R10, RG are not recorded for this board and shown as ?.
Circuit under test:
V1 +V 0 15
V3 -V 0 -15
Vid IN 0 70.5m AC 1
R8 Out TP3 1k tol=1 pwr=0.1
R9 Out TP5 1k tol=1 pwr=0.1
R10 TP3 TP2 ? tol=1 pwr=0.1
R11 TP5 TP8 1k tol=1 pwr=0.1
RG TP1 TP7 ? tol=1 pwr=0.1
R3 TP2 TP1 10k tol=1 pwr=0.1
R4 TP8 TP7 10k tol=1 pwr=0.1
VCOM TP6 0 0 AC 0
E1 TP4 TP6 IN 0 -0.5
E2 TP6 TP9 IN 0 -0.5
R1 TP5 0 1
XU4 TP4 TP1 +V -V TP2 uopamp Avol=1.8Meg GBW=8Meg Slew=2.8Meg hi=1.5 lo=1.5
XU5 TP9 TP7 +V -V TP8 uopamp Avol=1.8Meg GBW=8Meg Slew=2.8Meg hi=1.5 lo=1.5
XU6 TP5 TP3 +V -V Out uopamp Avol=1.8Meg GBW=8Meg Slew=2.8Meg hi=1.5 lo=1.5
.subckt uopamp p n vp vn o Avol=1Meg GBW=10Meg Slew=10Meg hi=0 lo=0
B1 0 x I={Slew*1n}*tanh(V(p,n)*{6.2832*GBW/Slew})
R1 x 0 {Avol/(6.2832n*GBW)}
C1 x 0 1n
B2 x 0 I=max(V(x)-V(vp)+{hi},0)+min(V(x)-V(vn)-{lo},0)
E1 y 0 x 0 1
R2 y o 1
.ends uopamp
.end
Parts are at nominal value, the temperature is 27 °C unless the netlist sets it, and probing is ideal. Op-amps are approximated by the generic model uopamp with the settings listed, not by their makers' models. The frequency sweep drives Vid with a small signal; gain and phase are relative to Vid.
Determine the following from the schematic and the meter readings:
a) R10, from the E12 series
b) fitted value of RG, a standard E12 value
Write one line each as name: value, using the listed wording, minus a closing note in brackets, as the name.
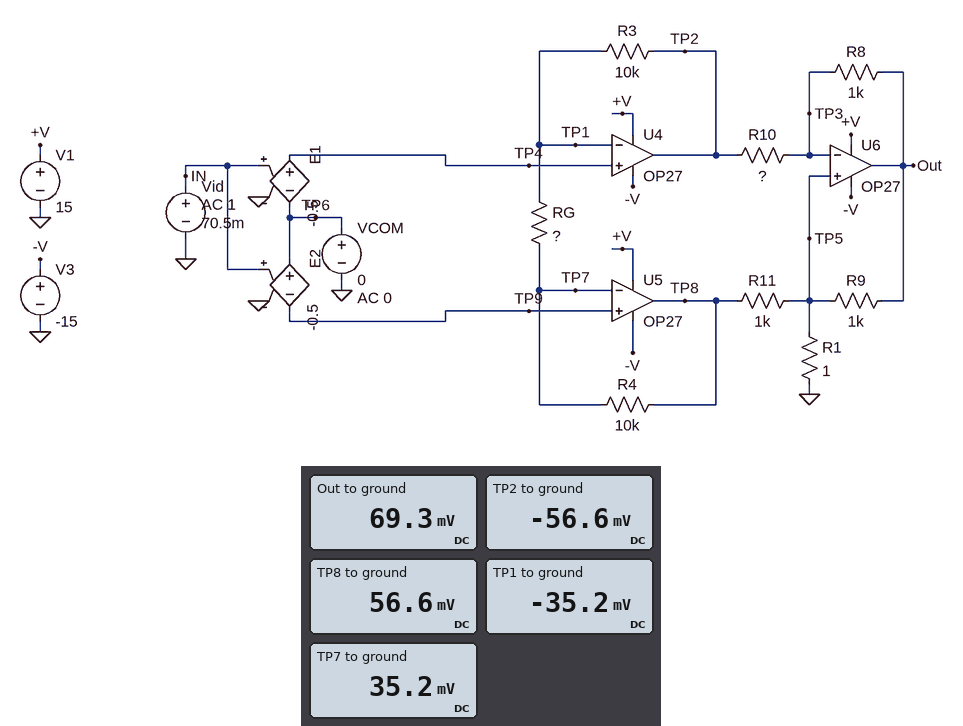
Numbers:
R10, from the E12 series: 820 Ω
fitted value of RG, a standard E12 value: 33 kΩ
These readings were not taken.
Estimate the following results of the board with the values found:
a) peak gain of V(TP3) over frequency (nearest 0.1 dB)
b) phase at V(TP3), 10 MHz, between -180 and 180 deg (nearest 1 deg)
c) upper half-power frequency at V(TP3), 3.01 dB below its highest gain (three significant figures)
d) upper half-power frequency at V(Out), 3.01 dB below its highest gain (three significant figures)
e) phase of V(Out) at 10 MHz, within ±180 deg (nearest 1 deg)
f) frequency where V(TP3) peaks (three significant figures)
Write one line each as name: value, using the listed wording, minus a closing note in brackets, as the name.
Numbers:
peak gain of V(TP3) over frequency: -11.8 dB
phase at V(TP3), 10 MHz, between -180 and 180 deg: 136 deg
upper half-power frequency at V(TP3), 3.01 dB below its highest gain: 10.3 MHz
upper half-power frequency at V(Out), 3.01 dB below its highest gain: 2.67 MHz
phase of V(Out) at 10 MHz, within ±180 deg: -134 deg
frequency where V(TP3) peaks: 4.23 MHz
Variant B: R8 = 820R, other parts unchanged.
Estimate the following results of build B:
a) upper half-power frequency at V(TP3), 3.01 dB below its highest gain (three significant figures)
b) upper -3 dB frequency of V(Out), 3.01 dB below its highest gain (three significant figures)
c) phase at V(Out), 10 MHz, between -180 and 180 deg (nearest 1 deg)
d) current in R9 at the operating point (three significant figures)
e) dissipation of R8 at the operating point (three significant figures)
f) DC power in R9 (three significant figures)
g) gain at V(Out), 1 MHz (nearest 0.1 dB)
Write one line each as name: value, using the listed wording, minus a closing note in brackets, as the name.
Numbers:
upper half-power frequency at V(TP3), 3.01 dB below its highest gain: 10.8 MHz
upper -3 dB frequency of V(Out), 3.01 dB below its highest gain: 2.84 MHz
phase at V(Out), 10 MHz, between -180 and 180 deg: -132 deg
current in R9 at the operating point: 56.7 µA
dissipation of R8 at the operating point: 3.92 µW
DC power in R9: 3.22 µW
gain at V(Out), 1 MHz: -2.3 dB
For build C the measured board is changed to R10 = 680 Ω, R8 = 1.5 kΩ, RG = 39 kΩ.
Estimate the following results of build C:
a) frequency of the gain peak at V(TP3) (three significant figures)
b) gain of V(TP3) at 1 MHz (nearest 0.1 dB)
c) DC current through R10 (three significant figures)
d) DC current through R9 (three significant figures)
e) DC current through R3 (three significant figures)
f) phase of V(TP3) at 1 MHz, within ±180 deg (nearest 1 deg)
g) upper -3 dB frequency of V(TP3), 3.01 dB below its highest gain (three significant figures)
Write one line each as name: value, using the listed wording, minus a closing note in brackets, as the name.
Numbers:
frequency of the gain peak at V(TP3): 3.62 MHz
gain of V(TP3) at 1 MHz: -14.4 dB
DC current through R10: 78.7 µA
DC current through R9: 118 µA
DC current through R3: 1.81 µA
phase of V(TP3) at 1 MHz, within ±180 deg: -122 deg
upper -3 dB frequency of V(TP3), 3.01 dB below its highest gain: 9.20 MHz
